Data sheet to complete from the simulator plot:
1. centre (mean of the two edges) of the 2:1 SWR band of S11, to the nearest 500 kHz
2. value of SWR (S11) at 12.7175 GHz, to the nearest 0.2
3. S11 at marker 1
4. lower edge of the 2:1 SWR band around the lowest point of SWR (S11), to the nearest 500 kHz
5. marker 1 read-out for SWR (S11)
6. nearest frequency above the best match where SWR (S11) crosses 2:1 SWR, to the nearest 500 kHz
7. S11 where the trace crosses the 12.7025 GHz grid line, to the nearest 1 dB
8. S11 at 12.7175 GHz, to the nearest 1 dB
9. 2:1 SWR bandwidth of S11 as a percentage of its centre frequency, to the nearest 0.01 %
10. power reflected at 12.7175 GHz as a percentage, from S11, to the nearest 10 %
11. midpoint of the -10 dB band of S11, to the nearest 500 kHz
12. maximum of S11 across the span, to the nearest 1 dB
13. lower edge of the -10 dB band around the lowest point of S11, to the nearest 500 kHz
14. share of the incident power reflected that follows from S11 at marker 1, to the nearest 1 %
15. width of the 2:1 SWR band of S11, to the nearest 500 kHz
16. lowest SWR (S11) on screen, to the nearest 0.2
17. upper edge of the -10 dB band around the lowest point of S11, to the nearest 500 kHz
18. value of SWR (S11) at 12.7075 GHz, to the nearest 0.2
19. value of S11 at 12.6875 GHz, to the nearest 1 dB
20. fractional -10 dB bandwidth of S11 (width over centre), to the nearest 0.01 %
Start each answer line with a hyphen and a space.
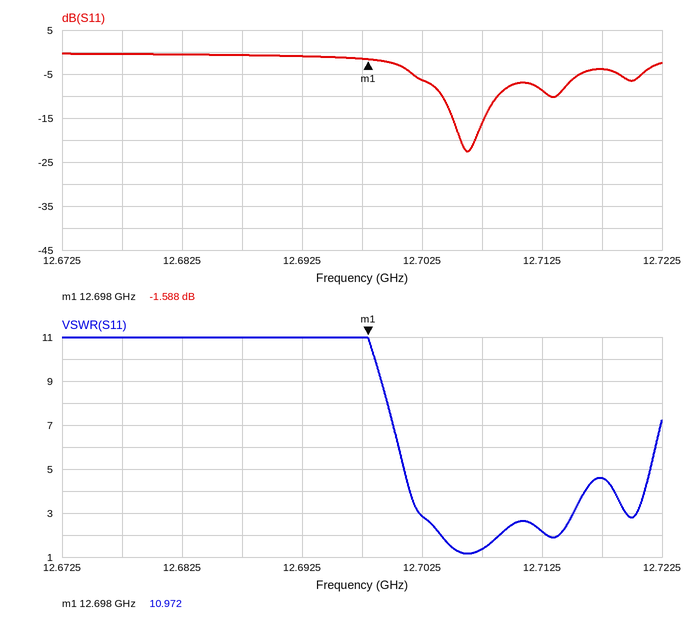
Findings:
- 12.7065 GHz
- 4.6
- -1.588 dB
- 12.7040 GHz
- 10.972
- 12.7090 GHz
- -6 dB
- -4 dB
- 0.04 %
- 40 %
- 12.7065 GHz
- 0 dB
- 12.7040 GHz
- 69 %
- 5.0 MHz
- 1.2
- 12.7090 GHz
- 1.4
- -1 dB
- 0.04 %
